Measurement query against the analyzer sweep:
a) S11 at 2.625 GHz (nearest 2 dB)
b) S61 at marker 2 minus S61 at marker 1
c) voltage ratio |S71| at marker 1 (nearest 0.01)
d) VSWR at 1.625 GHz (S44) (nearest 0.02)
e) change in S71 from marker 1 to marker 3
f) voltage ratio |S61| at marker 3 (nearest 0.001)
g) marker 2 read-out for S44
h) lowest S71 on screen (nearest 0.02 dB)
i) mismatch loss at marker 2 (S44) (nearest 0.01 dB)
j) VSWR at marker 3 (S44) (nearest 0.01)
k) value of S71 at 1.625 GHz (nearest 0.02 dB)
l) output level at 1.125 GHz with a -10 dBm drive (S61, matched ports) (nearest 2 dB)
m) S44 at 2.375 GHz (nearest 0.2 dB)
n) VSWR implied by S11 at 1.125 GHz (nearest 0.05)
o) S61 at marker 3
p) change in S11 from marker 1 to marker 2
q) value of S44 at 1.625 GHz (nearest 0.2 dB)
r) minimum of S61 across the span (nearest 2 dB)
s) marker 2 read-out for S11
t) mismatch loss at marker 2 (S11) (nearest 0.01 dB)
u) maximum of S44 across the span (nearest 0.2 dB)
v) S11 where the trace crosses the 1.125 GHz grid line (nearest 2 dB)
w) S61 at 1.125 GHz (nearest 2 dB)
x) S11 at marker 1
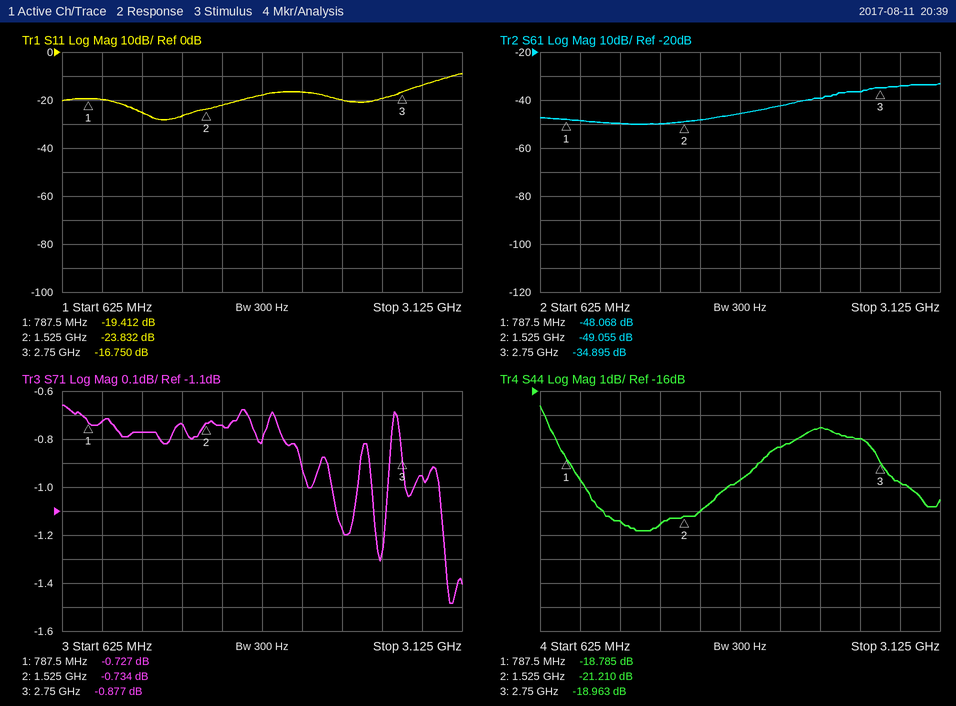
-20 dB
-0.987 dB
0.92
1.20
-0.150 dB
0.018
-21.210 dB
-1.48 dB
0.03 dB
1.25
-0.74 dB
-60 dBm
-17.6 dB
1.10
-34.895 dB
-4.420 dB
-21.0 dB
-50 dB
-23.832 dB
0.02 dB
-16.6 dB
-26 dB
-50 dB
-19.412 dB
